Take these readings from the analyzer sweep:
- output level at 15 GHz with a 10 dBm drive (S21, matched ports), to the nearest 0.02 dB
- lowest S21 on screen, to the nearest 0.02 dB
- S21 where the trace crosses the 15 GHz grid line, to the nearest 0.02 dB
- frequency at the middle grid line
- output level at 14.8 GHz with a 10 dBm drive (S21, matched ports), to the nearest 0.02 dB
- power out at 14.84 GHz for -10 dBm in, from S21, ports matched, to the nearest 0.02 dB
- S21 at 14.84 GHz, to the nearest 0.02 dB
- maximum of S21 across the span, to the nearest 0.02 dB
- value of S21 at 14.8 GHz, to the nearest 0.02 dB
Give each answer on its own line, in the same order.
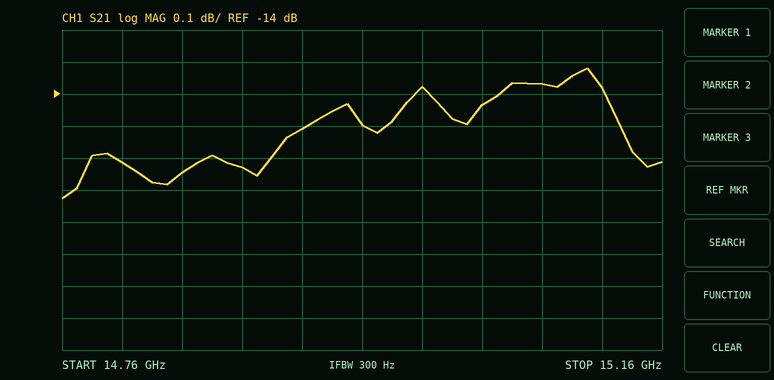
-3.98 dBm
-14.32 dB
-13.98 dB
14.96 GHz
-4.22 dBm
-24.24 dBm
-14.24 dB
-13.92 dB
-14.22 dB
